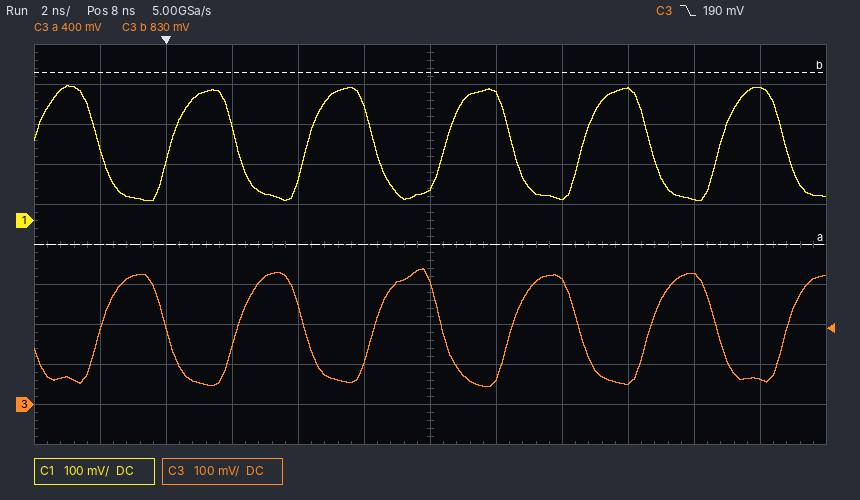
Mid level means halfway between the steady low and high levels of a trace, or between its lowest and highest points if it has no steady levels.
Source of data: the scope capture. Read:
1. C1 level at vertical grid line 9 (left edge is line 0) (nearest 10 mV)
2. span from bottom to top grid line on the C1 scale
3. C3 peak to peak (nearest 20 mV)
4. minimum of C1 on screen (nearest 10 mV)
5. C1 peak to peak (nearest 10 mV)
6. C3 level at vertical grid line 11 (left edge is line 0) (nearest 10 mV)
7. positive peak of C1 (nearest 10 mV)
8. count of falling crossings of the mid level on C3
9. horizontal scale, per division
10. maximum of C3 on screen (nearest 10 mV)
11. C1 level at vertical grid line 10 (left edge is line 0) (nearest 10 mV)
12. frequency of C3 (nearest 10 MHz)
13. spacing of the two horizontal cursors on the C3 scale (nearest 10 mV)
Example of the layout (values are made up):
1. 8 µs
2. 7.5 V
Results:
1. 330 mV
2. 1 V
3. 300 mV
4. 50 mV
5. 290 mV
6. 60 mV
7. 340 mV
8. 5
9. 2 ns
10. 340 mV
11. 50 mV
12. 240 MHz
13. 430 mV
